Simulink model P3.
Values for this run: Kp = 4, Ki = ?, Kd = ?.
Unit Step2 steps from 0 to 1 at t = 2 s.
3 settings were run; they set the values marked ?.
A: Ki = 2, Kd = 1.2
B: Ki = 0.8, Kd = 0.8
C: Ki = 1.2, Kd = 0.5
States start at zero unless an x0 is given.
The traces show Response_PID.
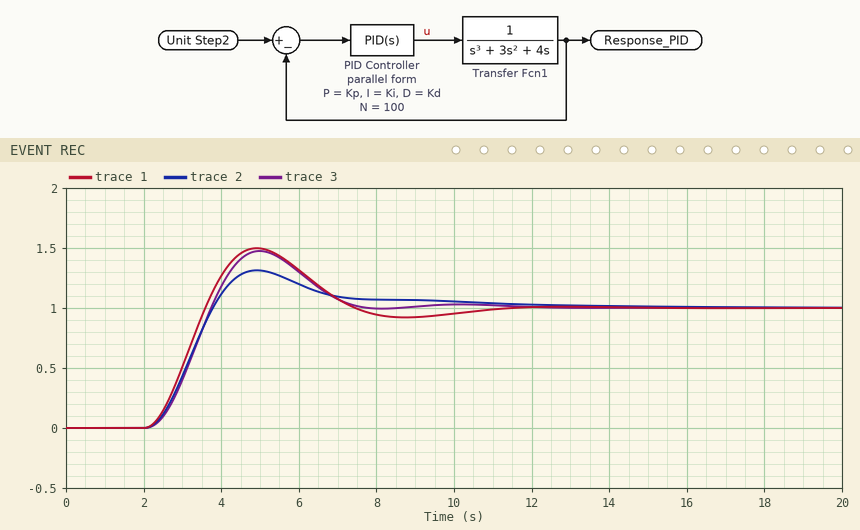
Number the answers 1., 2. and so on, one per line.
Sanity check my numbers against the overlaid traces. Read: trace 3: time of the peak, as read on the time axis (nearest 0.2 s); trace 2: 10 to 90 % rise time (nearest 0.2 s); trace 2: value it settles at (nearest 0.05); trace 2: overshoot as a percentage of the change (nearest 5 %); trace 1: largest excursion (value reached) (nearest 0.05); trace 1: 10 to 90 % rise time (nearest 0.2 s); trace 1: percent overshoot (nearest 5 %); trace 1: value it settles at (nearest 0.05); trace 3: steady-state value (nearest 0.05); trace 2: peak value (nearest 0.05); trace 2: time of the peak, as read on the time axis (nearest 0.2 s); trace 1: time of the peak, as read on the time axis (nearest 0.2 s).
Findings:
1. 5.0 s
2. 1.2 s
3. 1.00
4. 30 %
5. 1.50
6. 1.0 s
7. 50 %
8. 1.00
9. 1.00
10. 1.30
11. 5.0 s
12. 5.0 s
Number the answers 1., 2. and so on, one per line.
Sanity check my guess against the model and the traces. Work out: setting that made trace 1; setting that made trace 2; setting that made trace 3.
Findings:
1. A
2. B
3. C
